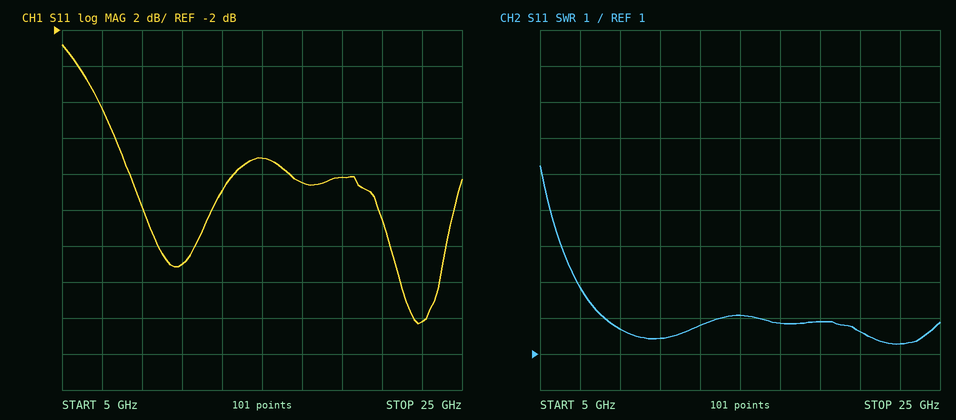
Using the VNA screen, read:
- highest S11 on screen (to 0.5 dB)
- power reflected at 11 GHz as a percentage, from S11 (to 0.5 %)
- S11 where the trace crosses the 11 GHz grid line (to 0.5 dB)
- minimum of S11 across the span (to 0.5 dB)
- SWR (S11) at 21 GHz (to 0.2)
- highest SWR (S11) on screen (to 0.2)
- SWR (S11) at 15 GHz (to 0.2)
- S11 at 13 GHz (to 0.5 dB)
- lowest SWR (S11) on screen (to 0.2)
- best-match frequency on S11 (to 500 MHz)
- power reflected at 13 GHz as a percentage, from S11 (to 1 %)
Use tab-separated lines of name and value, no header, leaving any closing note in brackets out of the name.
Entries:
highest S11 on screen	-3.0 dB
power reflected at 11 GHz as a percentage, from S11	3.0 %
S11 where the trace crosses the 11 GHz grid line	-15.0 dB
minimum of S11 across the span	-18.5 dB
SWR (S11) at 21 GHz	1.6
highest SWR (S11) on screen	6.2
SWR (S11) at 15 GHz	2.0
S11 at 13 GHz	-11.0 dB
lowest SWR (S11) on screen	1.2
best-match frequency on S11	23.0 GHz
power reflected at 13 GHz as a percentage, from S11	8 %
